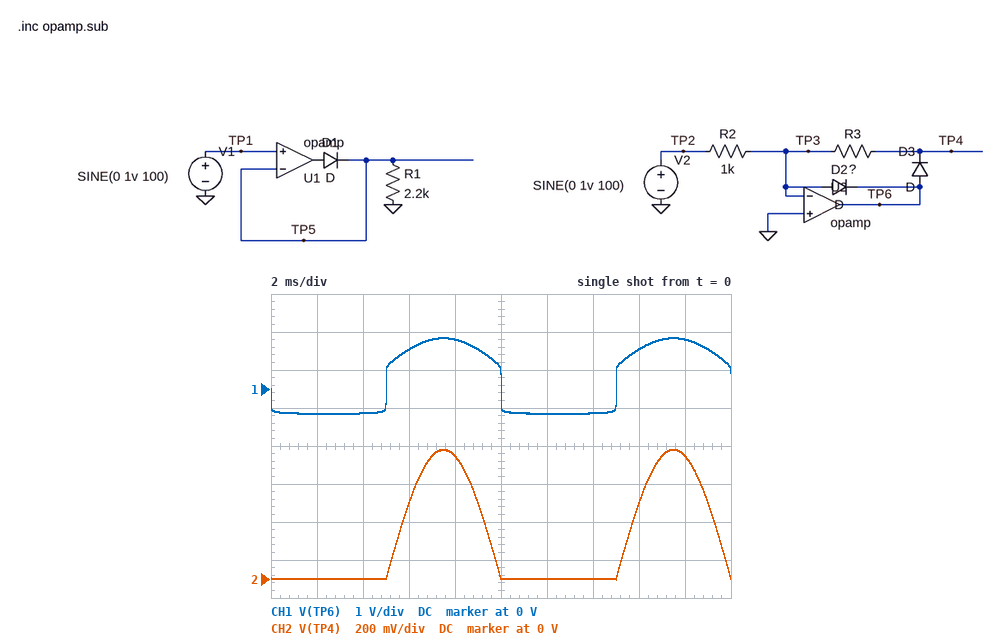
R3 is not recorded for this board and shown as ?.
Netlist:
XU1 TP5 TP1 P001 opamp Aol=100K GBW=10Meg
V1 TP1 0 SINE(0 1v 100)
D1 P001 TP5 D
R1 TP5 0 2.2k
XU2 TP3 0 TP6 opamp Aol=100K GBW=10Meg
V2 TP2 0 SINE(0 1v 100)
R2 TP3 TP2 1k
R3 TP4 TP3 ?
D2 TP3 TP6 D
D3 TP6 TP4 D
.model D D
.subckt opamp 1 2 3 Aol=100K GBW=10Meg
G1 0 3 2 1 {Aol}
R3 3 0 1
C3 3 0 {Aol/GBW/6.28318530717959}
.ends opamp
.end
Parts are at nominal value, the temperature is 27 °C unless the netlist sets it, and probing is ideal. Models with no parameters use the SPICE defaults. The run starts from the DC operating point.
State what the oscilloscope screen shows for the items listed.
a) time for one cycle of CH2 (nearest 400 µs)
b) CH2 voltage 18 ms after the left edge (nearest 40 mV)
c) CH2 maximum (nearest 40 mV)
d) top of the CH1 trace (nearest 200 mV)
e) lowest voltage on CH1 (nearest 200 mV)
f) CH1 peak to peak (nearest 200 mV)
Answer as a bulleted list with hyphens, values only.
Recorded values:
- 10.0 ms
- 640 mV
- 680 mV
- 1.4 V
- -600 mV
- 2.0 V
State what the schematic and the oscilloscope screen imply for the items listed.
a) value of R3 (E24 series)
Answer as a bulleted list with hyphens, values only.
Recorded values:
- 680 Ω
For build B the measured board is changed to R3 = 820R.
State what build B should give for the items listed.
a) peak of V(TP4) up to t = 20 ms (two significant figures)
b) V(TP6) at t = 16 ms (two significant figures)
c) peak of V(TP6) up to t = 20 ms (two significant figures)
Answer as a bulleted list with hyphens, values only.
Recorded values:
- 820 mV
- 1.1 V
- 1.5 V
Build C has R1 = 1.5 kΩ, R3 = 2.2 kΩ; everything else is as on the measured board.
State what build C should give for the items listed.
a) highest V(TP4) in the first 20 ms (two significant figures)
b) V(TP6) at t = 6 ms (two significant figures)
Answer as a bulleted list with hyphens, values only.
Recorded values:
- 2.2 V
- 1.9 V
